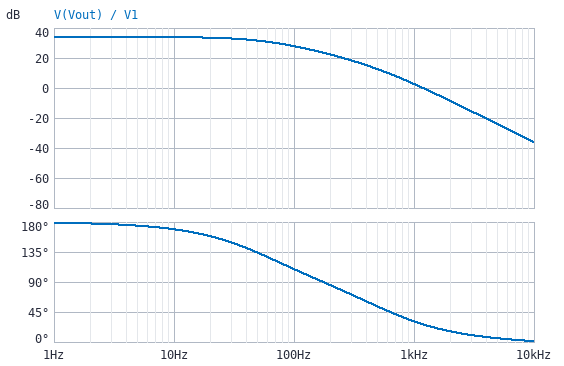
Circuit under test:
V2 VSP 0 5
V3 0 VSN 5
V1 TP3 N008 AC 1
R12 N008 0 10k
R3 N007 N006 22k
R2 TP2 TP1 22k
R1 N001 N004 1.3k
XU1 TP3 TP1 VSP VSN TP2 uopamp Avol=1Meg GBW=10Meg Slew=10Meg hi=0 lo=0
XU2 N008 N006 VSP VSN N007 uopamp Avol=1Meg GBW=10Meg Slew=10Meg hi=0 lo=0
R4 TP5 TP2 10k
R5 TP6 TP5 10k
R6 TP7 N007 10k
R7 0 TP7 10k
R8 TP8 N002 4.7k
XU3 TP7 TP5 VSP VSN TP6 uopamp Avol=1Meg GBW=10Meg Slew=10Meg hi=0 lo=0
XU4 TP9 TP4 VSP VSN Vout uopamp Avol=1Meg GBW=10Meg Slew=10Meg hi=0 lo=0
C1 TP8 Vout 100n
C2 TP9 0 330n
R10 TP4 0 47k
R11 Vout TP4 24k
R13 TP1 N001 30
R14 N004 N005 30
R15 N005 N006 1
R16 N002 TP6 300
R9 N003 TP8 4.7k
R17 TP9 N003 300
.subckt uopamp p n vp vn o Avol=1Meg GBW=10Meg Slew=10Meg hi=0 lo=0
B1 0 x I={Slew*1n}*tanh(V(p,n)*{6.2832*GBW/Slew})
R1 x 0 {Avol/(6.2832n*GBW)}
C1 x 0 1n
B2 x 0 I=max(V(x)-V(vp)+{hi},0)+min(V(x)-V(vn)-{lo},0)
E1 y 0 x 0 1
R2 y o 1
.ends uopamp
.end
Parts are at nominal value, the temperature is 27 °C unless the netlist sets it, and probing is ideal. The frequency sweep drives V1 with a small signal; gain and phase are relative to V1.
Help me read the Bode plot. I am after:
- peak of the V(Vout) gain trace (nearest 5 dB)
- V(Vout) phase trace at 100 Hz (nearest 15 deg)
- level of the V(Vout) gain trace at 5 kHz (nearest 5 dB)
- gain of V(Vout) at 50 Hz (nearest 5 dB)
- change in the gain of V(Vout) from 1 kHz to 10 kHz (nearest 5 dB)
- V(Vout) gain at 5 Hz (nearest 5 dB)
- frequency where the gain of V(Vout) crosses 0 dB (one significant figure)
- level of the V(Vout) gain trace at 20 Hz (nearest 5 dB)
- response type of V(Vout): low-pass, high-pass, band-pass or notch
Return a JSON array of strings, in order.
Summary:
["35 dB", "105 deg", "-25 dB", "30 dB", "-40 dB", "35 dB", "1 kHz", "35 dB", "low-pass"]
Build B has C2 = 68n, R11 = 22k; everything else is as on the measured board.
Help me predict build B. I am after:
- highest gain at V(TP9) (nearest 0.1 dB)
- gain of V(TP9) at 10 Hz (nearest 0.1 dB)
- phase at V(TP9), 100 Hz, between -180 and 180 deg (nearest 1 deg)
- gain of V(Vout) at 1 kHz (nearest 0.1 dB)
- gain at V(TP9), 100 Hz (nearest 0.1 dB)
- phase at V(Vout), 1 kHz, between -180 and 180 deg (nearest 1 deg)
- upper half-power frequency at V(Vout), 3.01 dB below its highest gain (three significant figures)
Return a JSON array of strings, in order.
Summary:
["31.3 dB", "30.5 dB", "163 deg", "17.7 dB", "30.7 dB", "26 deg", "444 Hz"]
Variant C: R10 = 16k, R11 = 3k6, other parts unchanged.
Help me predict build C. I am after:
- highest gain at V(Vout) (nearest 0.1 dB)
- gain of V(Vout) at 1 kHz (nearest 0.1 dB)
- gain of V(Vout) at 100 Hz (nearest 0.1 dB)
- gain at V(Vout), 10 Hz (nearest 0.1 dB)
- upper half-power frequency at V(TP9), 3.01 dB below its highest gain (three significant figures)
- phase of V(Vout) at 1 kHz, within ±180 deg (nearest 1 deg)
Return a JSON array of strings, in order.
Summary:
["32.2 dB", "0.8 dB", "25.7 dB", "32.1 dB", "54.3 Hz", "32 deg"]
